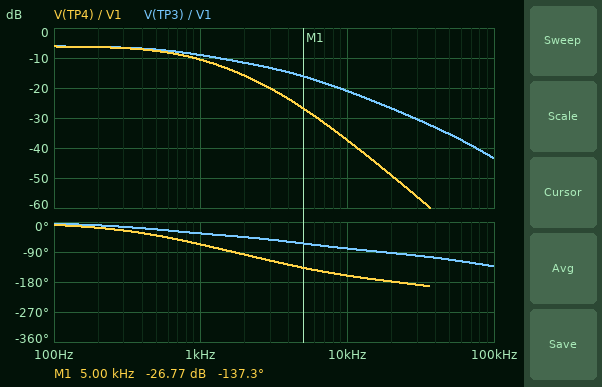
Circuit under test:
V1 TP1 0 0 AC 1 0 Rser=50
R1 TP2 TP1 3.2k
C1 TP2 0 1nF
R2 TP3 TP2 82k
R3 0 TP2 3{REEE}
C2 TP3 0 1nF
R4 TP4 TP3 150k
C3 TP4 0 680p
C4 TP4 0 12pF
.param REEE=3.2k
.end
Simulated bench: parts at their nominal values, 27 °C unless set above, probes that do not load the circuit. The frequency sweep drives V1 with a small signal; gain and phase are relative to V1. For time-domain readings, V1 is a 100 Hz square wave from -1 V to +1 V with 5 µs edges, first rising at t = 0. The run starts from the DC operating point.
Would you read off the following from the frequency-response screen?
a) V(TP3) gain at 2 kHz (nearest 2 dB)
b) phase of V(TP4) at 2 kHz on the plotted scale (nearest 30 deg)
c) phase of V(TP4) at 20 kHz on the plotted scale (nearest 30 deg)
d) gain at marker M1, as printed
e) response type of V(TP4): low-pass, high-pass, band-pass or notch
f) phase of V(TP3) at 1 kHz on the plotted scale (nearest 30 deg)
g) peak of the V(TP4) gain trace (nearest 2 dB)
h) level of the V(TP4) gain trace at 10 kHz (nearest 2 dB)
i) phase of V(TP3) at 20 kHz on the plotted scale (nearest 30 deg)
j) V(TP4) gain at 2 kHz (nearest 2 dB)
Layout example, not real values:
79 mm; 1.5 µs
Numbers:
-12 dB; -90 deg; -180 deg; -26.77 dB; low-pass; -30 deg; -6 dB; -38 dB; -90 deg; -16 dB
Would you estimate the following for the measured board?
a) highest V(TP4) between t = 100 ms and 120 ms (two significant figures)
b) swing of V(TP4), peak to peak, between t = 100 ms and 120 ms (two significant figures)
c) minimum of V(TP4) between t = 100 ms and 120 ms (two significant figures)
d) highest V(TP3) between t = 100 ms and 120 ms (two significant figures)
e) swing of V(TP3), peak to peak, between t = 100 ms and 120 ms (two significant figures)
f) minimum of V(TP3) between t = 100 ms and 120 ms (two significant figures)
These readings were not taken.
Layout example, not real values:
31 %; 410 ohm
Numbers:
500 mV; 990 mV; -500 mV; 500 mV; 990 mV; -500 mV
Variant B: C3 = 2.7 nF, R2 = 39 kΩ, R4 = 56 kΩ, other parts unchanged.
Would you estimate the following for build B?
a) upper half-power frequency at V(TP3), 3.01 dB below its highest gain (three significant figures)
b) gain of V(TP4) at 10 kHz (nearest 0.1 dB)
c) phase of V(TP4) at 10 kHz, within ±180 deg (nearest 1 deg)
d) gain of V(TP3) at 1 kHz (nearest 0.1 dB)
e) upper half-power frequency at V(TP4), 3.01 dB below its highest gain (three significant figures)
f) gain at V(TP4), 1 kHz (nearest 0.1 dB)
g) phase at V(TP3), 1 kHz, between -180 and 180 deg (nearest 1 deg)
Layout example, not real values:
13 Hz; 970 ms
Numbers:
860 Hz; -35.7 dB; -146 deg; -9.5 dB; 564 Hz; -12.3 dB; -25 deg
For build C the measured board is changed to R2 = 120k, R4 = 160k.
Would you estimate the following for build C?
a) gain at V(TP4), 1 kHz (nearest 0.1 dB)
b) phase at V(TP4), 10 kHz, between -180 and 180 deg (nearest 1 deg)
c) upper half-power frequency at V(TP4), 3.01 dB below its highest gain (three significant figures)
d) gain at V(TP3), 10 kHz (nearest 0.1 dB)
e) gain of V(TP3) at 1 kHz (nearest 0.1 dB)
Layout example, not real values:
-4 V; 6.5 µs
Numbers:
-12.3 dB; -165 deg; 579 Hz; -24.1 dB; -10.6 dB
